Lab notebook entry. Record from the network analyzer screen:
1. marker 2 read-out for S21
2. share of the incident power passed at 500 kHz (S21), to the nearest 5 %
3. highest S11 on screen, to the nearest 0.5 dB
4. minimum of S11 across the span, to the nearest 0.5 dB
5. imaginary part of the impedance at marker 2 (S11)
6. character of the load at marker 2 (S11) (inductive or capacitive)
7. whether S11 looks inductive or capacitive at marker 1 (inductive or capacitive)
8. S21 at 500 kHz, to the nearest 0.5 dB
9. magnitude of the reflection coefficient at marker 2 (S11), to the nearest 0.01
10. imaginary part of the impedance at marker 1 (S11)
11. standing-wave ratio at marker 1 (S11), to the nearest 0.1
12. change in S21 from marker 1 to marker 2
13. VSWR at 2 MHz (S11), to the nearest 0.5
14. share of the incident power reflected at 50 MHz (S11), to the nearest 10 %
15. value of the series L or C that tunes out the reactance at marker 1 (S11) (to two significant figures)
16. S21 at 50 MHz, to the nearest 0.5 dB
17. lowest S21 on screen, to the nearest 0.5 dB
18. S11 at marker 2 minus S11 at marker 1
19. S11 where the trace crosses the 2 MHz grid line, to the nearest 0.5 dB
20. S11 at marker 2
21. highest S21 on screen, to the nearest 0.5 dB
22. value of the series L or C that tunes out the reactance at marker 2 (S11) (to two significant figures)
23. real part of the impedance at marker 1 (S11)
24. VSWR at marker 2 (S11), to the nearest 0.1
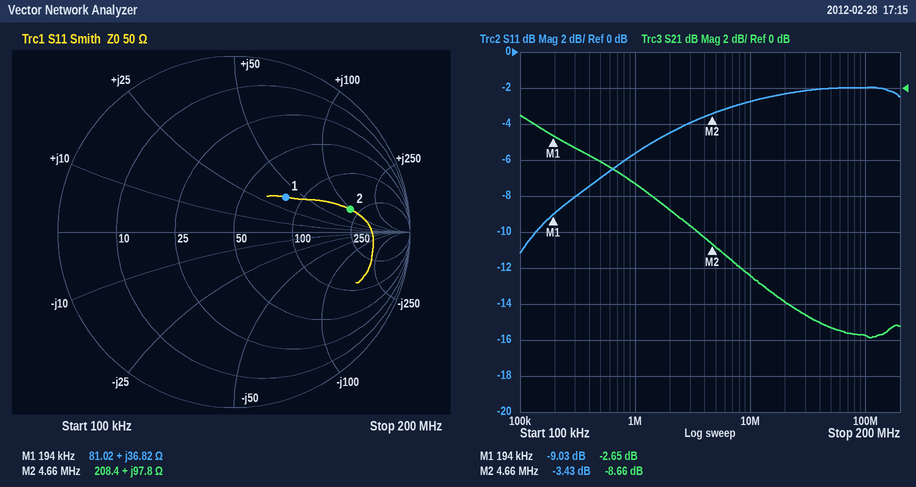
-8.66 dB
40 %
-2.0 dB
-11.0 dB
+97.8 Ω
inductive
inductive
-4.0 dB
0.67
+36.82 Ω
2.1
-6.01 dB
4.0
60 %
22 nF
-13.5 dB
-14.0 dB
5.60 dB
-4.5 dB
-3.43 dB
-1.5 dB
350 pF
81.02 Ω
5.1
